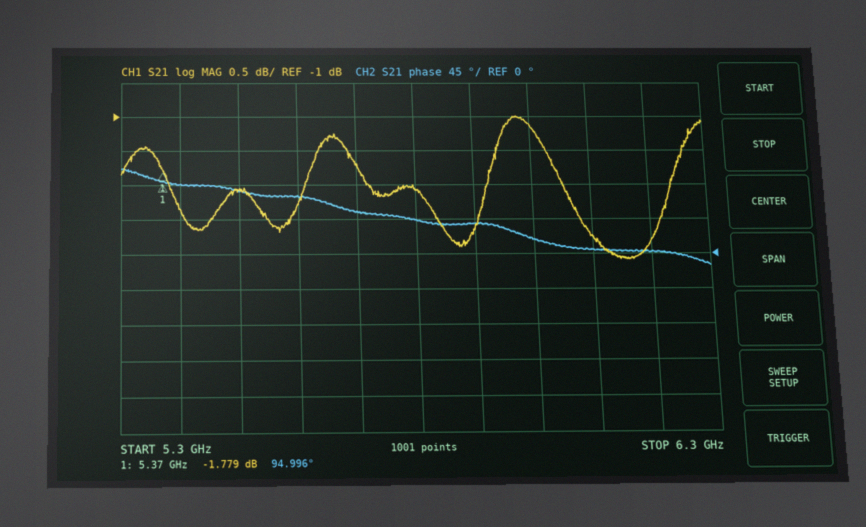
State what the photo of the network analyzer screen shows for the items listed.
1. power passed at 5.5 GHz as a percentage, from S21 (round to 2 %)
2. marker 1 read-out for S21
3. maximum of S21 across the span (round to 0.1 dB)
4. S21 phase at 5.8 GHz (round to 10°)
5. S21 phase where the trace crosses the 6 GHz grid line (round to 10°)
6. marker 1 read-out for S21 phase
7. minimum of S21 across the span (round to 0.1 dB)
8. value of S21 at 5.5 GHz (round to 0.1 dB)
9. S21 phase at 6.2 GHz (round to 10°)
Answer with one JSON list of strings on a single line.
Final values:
["62 %", "-1.779 dB", "-1.0 dB", "40°", "20°", "94.996°", "-3.1 dB", "-2.1 dB", "0°"]
